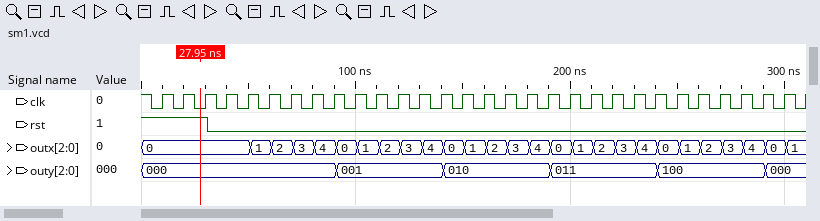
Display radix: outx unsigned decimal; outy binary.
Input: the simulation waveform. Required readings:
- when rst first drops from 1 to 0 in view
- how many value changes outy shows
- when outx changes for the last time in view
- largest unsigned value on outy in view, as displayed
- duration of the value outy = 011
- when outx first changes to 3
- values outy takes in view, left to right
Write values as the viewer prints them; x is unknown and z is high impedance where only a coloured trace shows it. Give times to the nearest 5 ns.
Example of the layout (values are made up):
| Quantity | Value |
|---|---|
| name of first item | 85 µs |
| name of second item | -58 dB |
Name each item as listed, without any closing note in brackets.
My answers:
| Quantity | Value |
|---|---|
| when rst first drops from 1 to 0 in view | 30 ns |
| how many value changes outy shows | 5 |
| when outx changes for the last time in view | 300 ns |
| largest unsigned value on outy in view, as displayed | 100 |
| duration of the value outy = 011 | 50 ns |
| when outx first changes to 3 | 70 ns |
| values outy takes in view, left to right | 000, 001, 010, 011, 100, 000 |
